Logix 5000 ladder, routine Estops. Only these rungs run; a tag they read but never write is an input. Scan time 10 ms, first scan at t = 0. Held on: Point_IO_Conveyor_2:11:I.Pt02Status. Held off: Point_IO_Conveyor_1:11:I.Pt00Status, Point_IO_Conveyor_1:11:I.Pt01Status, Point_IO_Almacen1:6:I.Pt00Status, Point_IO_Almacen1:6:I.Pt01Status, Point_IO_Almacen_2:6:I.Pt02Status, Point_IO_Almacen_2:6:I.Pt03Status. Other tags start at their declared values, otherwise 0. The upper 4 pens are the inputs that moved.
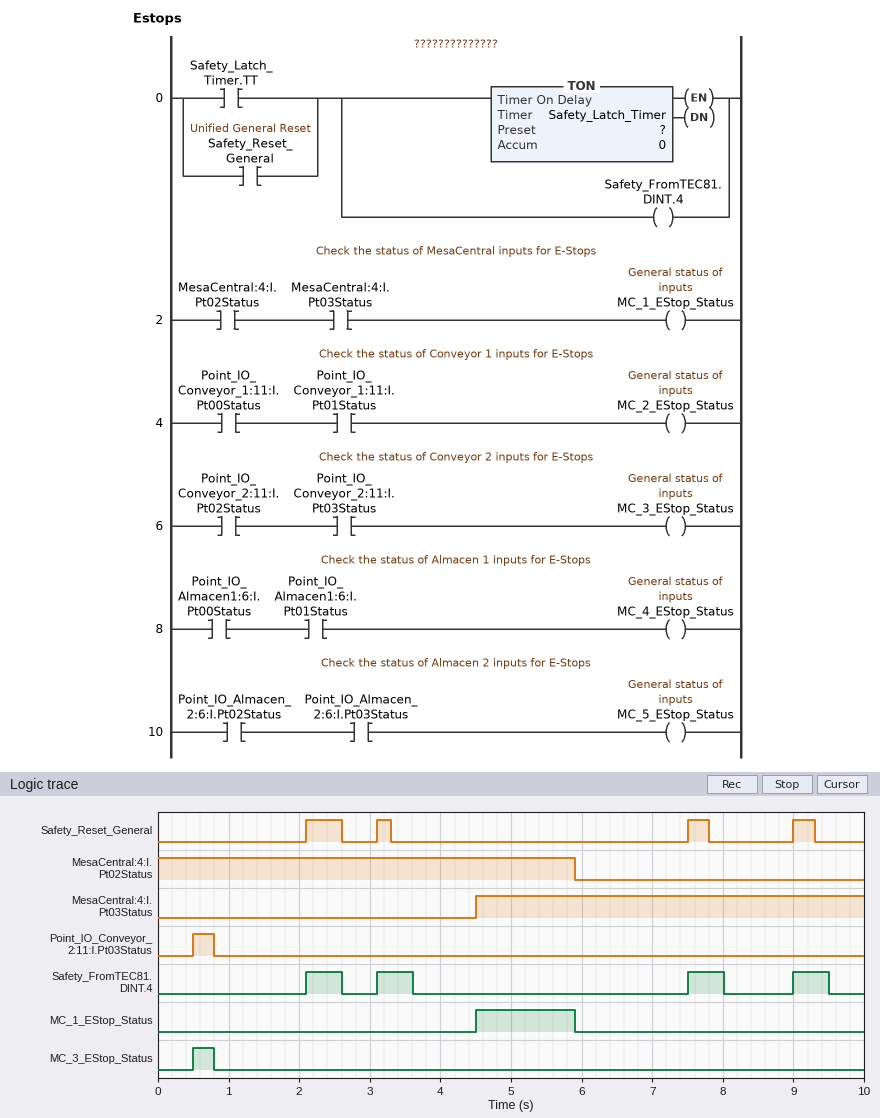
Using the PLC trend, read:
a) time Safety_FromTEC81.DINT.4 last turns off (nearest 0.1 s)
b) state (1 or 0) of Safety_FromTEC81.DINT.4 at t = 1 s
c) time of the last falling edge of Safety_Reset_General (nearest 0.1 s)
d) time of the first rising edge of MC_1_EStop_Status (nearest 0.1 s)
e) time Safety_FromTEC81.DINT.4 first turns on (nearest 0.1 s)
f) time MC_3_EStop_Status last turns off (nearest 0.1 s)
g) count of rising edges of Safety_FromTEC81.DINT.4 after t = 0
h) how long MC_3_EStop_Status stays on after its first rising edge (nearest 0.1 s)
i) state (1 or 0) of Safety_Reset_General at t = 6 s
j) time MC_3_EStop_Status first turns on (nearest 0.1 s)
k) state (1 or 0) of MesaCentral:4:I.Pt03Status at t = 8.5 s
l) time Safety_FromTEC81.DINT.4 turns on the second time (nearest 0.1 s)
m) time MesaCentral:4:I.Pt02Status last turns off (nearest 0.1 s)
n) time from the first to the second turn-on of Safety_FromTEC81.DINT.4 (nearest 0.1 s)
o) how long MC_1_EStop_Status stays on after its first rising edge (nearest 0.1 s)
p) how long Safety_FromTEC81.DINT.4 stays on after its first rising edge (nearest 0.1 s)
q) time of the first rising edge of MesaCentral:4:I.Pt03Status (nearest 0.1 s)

9.5 s
0
9.3 s
4.5 s
2.1 s
0.8 s
4
0.3 s
0
0.5 s
1
3.1 s
5.9 s
1.0 s
1.4 s
0.5 s
4.5 s
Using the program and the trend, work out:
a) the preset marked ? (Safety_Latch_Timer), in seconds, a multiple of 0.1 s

0.5 s
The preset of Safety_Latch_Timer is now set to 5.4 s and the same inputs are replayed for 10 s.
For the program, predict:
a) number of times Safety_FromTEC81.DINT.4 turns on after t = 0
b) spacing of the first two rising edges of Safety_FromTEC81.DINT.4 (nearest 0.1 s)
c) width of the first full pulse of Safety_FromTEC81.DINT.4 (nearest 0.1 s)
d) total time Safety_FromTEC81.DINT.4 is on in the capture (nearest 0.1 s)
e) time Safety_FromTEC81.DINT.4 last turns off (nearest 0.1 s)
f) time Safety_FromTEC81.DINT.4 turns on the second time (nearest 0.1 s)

2
6.9 s
5.7 s
6.7 s
7.8 s
9.0 s
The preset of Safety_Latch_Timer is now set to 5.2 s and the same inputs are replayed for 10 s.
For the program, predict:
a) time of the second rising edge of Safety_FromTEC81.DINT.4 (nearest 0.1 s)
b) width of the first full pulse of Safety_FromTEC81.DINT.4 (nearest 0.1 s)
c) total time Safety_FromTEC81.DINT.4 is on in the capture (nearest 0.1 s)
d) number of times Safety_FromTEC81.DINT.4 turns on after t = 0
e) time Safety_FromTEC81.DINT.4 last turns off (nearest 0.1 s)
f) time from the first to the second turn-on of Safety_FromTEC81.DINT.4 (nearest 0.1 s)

7.5 s
5.2 s
7.7 s
2
7.3 s
5.4 s
